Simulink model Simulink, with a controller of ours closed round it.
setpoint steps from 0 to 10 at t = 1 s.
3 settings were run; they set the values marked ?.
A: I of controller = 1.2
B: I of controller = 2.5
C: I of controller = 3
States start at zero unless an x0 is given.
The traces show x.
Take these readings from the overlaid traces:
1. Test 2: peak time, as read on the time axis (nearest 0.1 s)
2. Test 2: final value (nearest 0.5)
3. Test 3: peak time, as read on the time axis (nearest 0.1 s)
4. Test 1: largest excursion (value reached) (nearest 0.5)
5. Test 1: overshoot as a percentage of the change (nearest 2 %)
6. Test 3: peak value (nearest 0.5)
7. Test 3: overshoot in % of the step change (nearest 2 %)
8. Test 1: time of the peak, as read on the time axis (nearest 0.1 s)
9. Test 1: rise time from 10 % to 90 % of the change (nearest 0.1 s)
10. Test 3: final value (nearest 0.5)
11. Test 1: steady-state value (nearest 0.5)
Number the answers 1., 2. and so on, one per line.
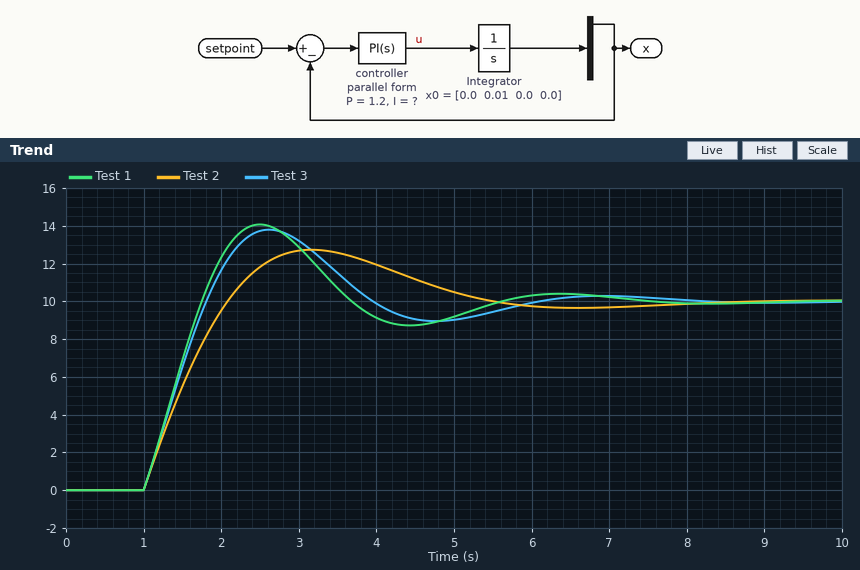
1. 3.2 s
2. 10.0
3. 2.6 s
4. 14.0
5. 40 %
6. 14.0
7. 38 %
8. 2.5 s
9. 0.6 s
10. 10.0
11. 10.0
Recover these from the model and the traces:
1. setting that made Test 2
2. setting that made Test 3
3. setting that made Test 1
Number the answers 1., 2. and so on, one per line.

1. A
2. B
3. C
